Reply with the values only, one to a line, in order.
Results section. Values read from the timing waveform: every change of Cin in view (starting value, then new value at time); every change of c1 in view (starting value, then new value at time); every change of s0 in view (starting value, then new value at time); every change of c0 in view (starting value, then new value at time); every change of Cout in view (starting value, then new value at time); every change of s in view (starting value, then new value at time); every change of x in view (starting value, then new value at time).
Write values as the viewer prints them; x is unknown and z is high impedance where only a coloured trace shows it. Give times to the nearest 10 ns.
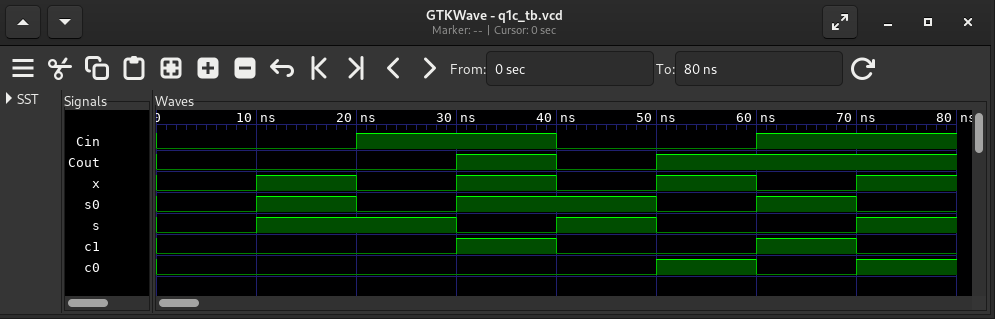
0, 1 at 20 ns, 0 at 40 ns, 1 at 60 ns
0, 1 at 30 ns, 0 at 40 ns, 1 at 60 ns, 0 at 70 ns
0, 1 at 10 ns, 0 at 20 ns, 1 at 30 ns, 0 at 50 ns, 1 at 60 ns, 0 at 70 ns
0, 1 at 50 ns, 0 at 60 ns, 1 at 70 ns
0, 1 at 30 ns, 0 at 40 ns, 1 at 50 ns
0, 1 at 10 ns, 0 at 30 ns, 1 at 40 ns, 0 at 50 ns, 1 at 70 ns
0, 1 at 10 ns, 0 at 20 ns, 1 at 30 ns, 0 at 40 ns, 1 at 50 ns, 0 at 60 ns, 1 at 70 ns
